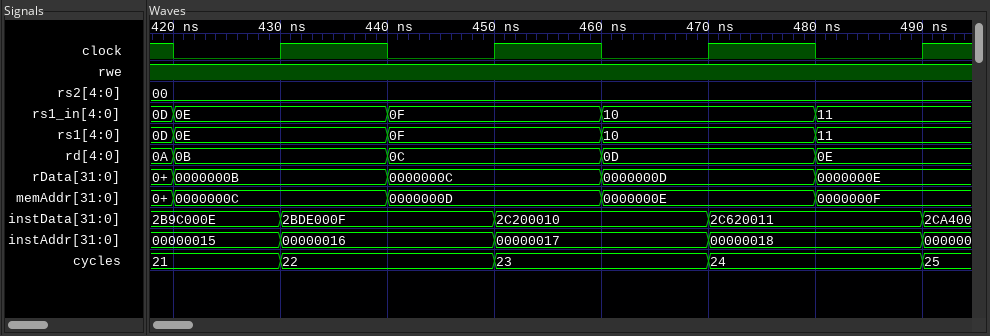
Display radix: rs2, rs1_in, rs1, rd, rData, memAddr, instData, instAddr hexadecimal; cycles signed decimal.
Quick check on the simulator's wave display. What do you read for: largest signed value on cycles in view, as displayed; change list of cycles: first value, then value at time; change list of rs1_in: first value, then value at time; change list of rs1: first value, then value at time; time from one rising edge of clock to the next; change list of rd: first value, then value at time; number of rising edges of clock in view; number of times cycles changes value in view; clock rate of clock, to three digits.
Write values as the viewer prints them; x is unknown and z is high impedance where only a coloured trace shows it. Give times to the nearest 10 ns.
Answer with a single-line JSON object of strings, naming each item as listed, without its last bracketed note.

{"largest signed value on cycles in view, as displayed": "25", "change list of cycles: first value, then value at time": "21, 22 at 430 ns, 23 at 450 ns, 24 at 470 ns, 25 at 490 ns", "change list of rs1_in: first value, then value at time": "0D, 0E at 420 ns, 0F at 440 ns, 10 at 460 ns, 11 at 480 ns", "change list of rs1: first value, then value at time": "0D, 0E at 420 ns, 0F at 440 ns, 10 at 460 ns, 11 at 480 ns", "time from one rising edge of clock to the next": "20 ns", "change list of rd: first value, then value at time": "0A, 0B at 420 ns, 0C at 440 ns, 0D at 460 ns, 0E at 480 ns", "number of rising edges of clock in view": "4", "number of times cycles changes value in view": "4", "clock rate of clock, to three digits": "50.0 MHz"}
